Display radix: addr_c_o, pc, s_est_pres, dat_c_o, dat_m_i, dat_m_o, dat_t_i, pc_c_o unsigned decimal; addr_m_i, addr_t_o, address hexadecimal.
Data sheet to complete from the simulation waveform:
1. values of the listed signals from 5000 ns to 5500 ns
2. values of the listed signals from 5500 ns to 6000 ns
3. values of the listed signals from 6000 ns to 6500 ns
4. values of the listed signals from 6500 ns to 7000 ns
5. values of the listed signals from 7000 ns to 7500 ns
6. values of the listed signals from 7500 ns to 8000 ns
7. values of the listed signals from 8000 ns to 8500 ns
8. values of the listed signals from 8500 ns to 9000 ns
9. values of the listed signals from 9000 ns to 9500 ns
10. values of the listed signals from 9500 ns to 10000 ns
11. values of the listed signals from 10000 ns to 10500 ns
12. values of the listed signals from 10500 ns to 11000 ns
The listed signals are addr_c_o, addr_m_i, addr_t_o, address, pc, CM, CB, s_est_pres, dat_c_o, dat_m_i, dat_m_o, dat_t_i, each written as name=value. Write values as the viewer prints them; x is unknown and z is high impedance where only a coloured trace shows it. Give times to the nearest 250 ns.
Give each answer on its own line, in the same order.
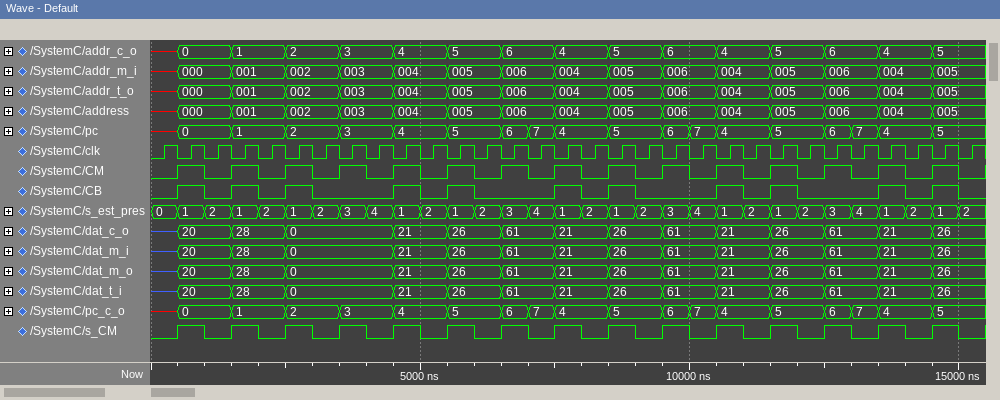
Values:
addr_c_o=4, addr_m_i=004, addr_t_o=004, address=004, pc=4, CM=0, CB=0, s_est_pres=2, dat_c_o=21, dat_m_i=21, dat_m_o=21, dat_t_i=21
addr_c_o=5, addr_m_i=005, addr_t_o=005, address=005, pc=5, CM=1, CB=1, s_est_pres=1, dat_c_o=26, dat_m_i=26, dat_m_o=26, dat_t_i=26
addr_c_o=5, addr_m_i=005, addr_t_o=005, address=005, pc=5, CM=0, CB=0, s_est_pres=2, dat_c_o=26, dat_m_i=26, dat_m_o=26, dat_t_i=26
addr_c_o=6, addr_m_i=006, addr_t_o=006, address=006, pc=6, CM=1, CB=0, s_est_pres=3, dat_c_o=61, dat_m_i=61, dat_m_o=61, dat_t_i=61
addr_c_o=6, addr_m_i=006, addr_t_o=006, address=006, pc=7, CM=0, CB=0, s_est_pres=4, dat_c_o=61, dat_m_i=61, dat_m_o=61, dat_t_i=61
addr_c_o=4, addr_m_i=004, addr_t_o=004, address=004, pc=4, CM=1, CB=1, s_est_pres=1, dat_c_o=21, dat_m_i=21, dat_m_o=21, dat_t_i=21
addr_c_o=4, addr_m_i=004, addr_t_o=004, address=004, pc=4, CM=0, CB=0, s_est_pres=2, dat_c_o=21, dat_m_i=21, dat_m_o=21, dat_t_i=21
addr_c_o=5, addr_m_i=005, addr_t_o=005, address=005, pc=5, CM=1, CB=1, s_est_pres=1, dat_c_o=26, dat_m_i=26, dat_m_o=26, dat_t_i=26
addr_c_o=5, addr_m_i=005, addr_t_o=005, address=005, pc=5, CM=0, CB=0, s_est_pres=2, dat_c_o=26, dat_m_i=26, dat_m_o=26, dat_t_i=26
addr_c_o=6, addr_m_i=006, addr_t_o=006, address=006, pc=6, CM=1, CB=0, s_est_pres=3, dat_c_o=61, dat_m_i=61, dat_m_o=61, dat_t_i=61
addr_c_o=6, addr_m_i=006, addr_t_o=006, address=006, pc=7, CM=0, CB=0, s_est_pres=4, dat_c_o=61, dat_m_i=61, dat_m_o=61, dat_t_i=61
addr_c_o=4, addr_m_i=004, addr_t_o=004, address=004, pc=4, CM=1, CB=1, s_est_pres=1, dat_c_o=21, dat_m_i=21, dat_m_o=21, dat_t_i=21
